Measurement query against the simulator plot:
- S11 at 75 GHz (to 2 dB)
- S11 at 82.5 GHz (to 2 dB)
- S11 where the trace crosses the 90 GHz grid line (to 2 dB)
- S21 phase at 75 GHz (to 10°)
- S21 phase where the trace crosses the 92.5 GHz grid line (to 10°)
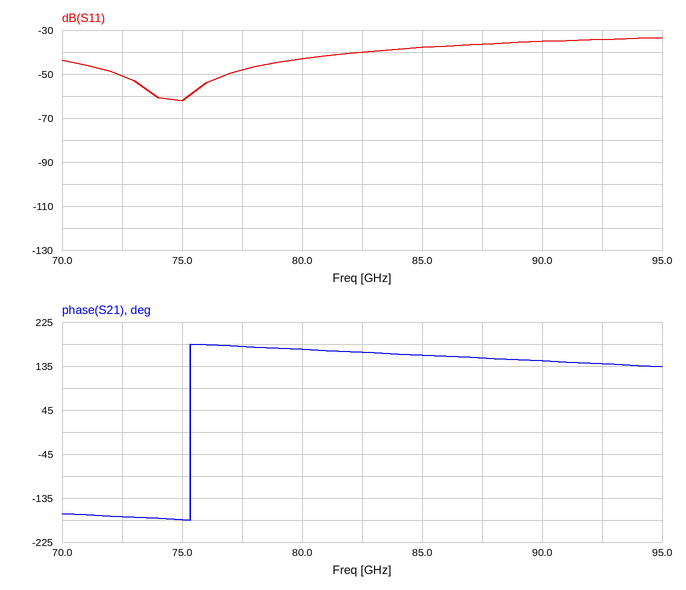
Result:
-62 dB
-40 dB
-36 dB
-180°
140°
